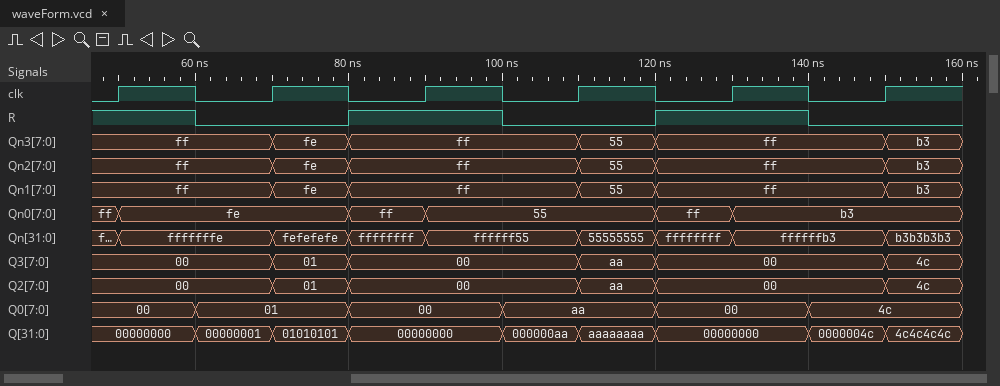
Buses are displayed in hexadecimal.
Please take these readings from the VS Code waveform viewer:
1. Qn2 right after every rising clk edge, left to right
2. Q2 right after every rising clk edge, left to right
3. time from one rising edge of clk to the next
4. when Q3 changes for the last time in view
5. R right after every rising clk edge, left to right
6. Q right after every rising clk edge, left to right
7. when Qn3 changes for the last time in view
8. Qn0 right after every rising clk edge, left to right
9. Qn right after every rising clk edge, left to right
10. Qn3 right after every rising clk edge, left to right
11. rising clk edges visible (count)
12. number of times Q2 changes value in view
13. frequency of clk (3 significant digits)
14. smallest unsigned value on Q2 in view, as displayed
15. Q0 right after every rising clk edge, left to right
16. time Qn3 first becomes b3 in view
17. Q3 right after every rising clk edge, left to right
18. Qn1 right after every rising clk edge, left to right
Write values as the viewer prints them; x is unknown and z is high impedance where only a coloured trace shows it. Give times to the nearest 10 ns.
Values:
ff, fe, ff, 55, ff, b3
00, 01, 00, aa, 00, 4c
20 ns
150 ns
1 0 1 0 1 0
00000000, 01010101, 00000000, aaaaaaaa, 00000000, 4c4c4c4c
150 ns
fe, fe, 55, 55, b3, b3
fffffffe, fefefefe, ffffff55, 55555555, ffffffb3, b3b3b3b3
ff, fe, ff, 55, ff, b3
6
5
50.0 MHz
00
00, 01, 00, aa, 00, 4c
150 ns
00, 01, 00, aa, 00, 4c
ff, fe, ff, 55, ff, b3
